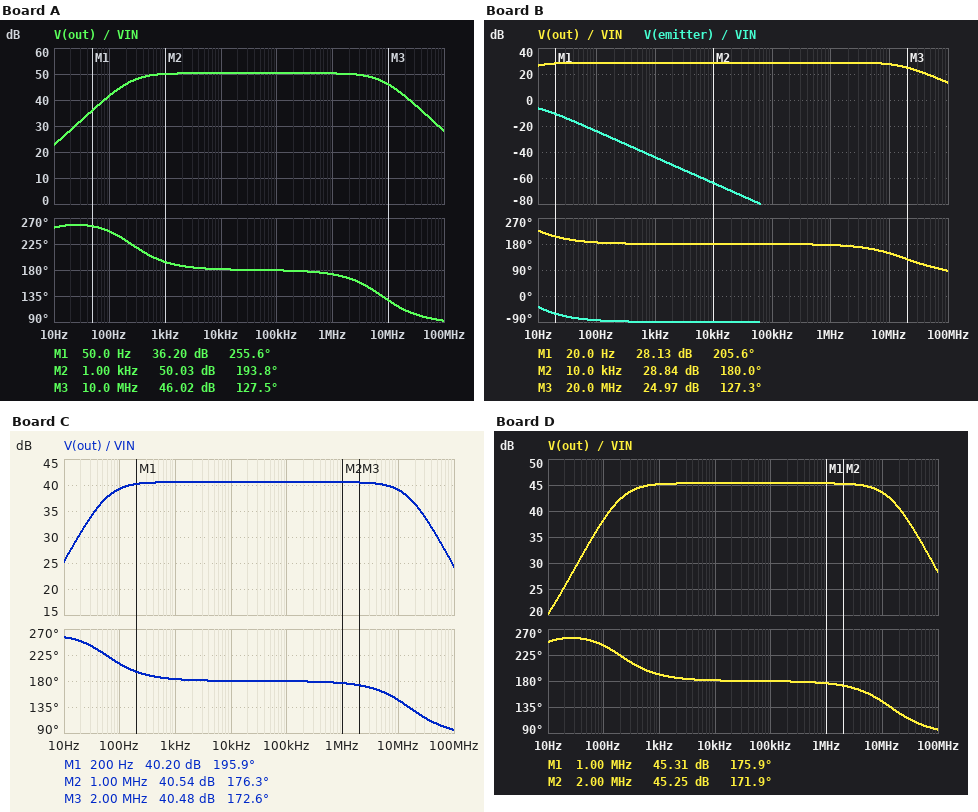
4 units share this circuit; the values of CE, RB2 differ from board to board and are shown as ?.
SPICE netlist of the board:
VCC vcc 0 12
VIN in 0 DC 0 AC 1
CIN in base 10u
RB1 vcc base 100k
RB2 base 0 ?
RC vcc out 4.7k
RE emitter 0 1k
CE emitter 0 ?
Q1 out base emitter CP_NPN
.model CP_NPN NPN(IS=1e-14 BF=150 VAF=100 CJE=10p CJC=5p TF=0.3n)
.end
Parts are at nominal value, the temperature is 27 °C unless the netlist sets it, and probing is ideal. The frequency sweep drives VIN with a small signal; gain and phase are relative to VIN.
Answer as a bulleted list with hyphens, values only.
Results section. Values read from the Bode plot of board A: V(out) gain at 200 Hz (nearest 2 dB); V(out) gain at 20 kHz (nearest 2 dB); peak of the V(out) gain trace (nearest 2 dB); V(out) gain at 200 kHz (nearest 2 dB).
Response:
- 46 dB
- 50 dB
- 50 dB
- 50 dB
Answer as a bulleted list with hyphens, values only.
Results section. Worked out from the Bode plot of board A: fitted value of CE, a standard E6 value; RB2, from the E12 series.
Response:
- 47 µF
- 33 kΩ
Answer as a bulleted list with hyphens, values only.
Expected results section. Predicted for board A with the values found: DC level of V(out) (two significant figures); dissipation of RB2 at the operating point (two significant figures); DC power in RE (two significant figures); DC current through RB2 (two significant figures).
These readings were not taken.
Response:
- 2.8 V
- 210 µW
- 3.9 mW
- 80 µA
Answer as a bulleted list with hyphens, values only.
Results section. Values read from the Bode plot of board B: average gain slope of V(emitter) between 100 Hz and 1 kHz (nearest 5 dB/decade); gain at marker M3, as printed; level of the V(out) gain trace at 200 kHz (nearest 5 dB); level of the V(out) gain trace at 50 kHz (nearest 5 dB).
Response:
- -20 dB/decade
- 24.97 dB
- 30 dB
- 30 dB
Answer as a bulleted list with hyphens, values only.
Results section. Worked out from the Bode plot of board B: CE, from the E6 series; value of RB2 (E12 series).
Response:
- 150 µF
- 6.8 kΩ
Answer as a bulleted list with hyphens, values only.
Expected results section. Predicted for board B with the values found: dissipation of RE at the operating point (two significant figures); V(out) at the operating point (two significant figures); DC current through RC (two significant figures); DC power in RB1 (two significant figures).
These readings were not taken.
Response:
- 24 µW
- 11 V
- 150 µA
- 1.3 mW
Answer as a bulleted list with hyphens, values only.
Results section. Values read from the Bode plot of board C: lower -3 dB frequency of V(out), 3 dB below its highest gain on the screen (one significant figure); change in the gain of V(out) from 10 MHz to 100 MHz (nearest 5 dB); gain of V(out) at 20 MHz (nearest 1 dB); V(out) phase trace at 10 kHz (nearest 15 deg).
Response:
- 60 Hz
- -15 dB
- 36 dB
- 180 deg
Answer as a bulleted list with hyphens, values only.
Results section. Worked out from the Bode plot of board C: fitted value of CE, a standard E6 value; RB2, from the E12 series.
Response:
- 68 µF
- 12 kΩ
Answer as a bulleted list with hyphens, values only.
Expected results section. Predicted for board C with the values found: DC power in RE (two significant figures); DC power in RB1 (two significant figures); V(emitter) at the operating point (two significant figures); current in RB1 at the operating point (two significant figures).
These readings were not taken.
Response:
- 370 µW
- 1.2 mW
- 610 mV
- 110 µA
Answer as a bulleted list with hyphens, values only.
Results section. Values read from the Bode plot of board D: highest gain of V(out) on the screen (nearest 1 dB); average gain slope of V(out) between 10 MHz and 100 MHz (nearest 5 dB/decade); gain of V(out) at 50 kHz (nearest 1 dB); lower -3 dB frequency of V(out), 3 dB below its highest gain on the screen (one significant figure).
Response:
- 45 dB
- -15 dB/decade
- 45 dB
- 200 Hz
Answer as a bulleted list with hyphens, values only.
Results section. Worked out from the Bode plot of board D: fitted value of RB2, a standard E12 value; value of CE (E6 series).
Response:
- 18 kΩ
- 33 µF
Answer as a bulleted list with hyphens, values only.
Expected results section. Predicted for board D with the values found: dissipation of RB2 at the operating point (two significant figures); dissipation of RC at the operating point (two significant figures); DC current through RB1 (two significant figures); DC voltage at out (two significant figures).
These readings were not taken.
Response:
- 170 µW
- 5.3 mW
- 100 µA
- 7.0 V
